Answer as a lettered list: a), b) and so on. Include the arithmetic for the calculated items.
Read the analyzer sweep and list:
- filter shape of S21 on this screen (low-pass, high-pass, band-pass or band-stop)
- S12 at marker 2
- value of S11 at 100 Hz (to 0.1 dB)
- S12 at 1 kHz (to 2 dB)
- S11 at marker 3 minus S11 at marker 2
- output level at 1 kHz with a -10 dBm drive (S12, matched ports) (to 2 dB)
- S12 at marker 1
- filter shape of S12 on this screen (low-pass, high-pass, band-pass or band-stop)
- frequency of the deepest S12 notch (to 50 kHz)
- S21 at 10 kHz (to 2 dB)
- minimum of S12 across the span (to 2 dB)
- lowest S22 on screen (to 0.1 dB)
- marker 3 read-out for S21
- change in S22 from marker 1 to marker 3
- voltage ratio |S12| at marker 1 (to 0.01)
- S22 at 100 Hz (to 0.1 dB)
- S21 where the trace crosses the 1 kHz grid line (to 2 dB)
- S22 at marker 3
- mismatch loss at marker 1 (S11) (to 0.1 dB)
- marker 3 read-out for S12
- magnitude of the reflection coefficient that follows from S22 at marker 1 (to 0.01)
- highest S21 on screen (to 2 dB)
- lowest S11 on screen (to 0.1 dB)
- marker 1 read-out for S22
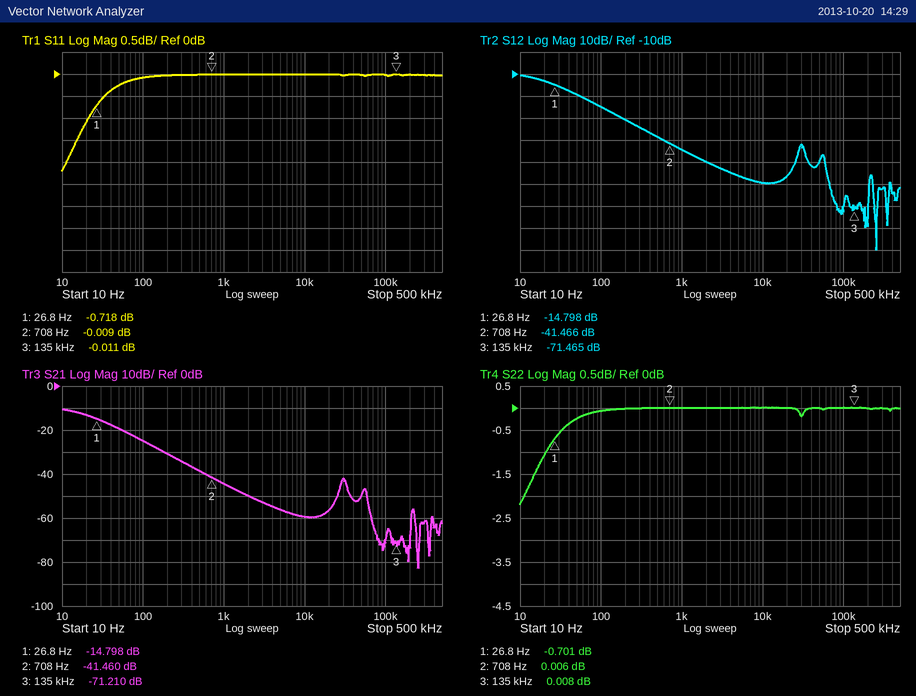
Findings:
a) low-pass
b) -41.466 dB
c) -0.1 dB
d) -44 dB
e) -0.011 − (-0.009) = -0.002 dB
f) -10 dBm + (-44 dB) = -54 dBm
g) -14.798 dB
h) low-pass
i) 250 kHz
j) -60 dB
k) -90 dB
l) -2.2 dB
m) -71.210 dB
n) 0.008 − (-0.701) = 0.709 dB
o) 10^(-14.798/20) ≈ 0.18
p) -0.1 dB
q) -44 dB
r) 0.008 dB
s) −10 log10(1 − 10^(-0.718/10)) ≈ 8.2 dB
t) -71.465 dB
u) 10^(-0.701/20) ≈ 0.92
v) -10 dB
w) -2.2 dB
x) -0.701 dB
